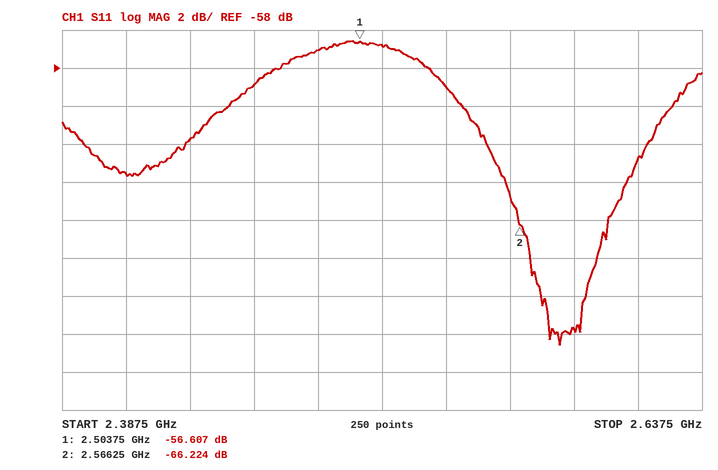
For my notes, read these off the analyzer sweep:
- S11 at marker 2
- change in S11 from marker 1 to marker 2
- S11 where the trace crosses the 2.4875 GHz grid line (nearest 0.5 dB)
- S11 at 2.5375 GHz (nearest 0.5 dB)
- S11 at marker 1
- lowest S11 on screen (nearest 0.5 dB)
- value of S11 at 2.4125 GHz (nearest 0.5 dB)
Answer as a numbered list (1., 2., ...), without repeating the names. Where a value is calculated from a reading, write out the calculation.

1. -66.224 dB
2. -66.224 − (-56.607) = -9.617 dB
3. -57.0 dB
4. -59.0 dB
5. -56.607 dB
6. -72.5 dB
7. -63.5 dB
